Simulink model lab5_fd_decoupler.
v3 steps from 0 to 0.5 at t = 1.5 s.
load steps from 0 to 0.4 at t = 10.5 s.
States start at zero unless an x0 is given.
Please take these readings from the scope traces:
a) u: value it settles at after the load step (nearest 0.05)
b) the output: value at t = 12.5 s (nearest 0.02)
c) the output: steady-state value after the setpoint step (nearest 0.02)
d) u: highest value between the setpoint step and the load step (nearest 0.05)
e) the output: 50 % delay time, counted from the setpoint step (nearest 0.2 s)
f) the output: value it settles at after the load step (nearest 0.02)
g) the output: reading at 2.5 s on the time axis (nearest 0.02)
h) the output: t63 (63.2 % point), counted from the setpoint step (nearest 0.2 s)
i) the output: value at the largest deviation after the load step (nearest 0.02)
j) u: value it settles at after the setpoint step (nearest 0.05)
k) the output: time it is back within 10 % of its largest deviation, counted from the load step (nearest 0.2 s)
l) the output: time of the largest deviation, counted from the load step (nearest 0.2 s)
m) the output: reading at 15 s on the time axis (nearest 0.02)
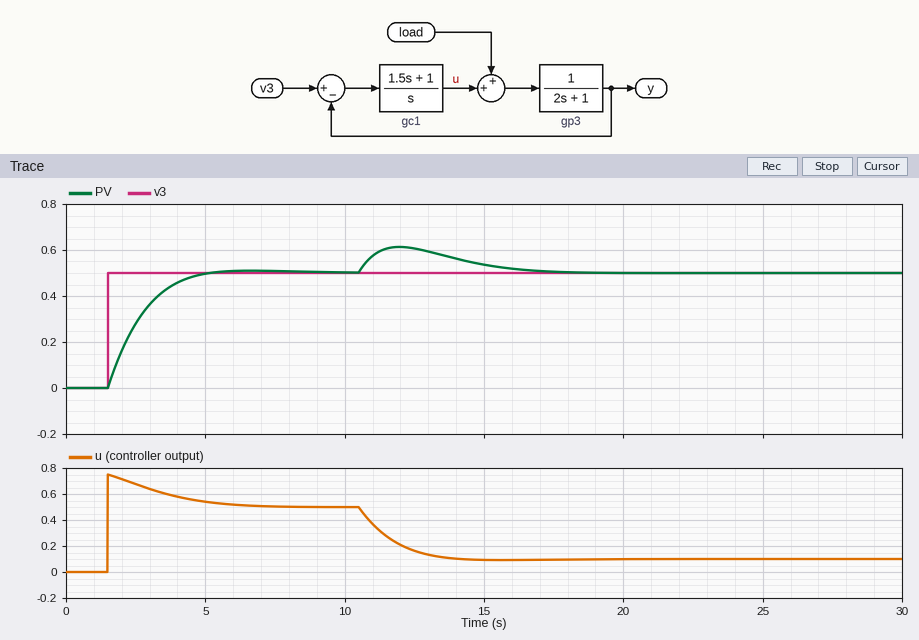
0.10
0.60
0.50
0.75
0.8 s
0.50
0.28
1.2 s
0.62
0.50
6.2 s
1.4 s
0.54
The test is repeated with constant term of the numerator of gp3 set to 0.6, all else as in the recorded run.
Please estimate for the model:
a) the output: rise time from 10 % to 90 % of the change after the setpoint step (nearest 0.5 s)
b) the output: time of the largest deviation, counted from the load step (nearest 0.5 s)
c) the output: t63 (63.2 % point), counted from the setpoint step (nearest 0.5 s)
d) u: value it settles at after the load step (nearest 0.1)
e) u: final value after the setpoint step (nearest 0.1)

3.5 s
2.0 s
2.0 s
0.4
0.8
